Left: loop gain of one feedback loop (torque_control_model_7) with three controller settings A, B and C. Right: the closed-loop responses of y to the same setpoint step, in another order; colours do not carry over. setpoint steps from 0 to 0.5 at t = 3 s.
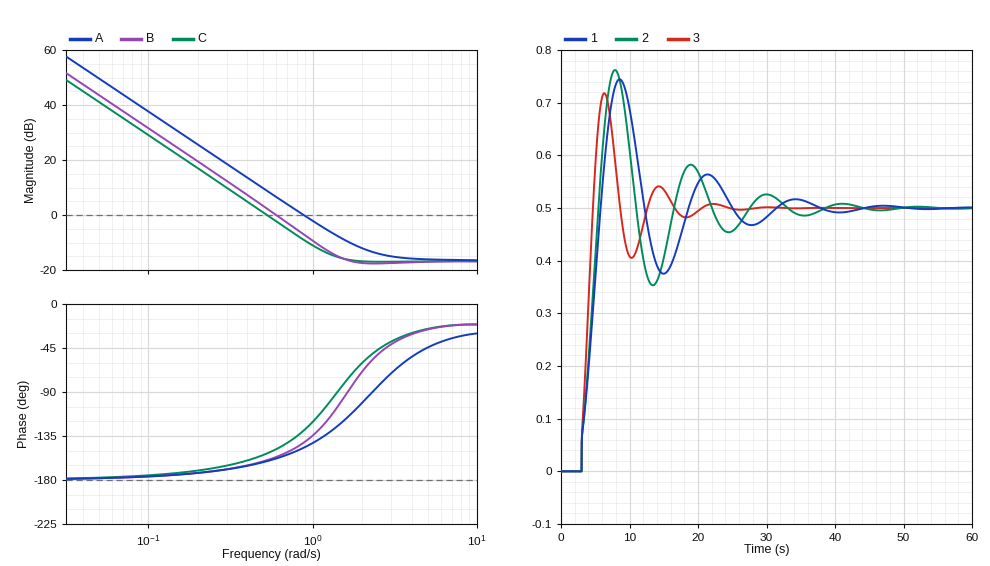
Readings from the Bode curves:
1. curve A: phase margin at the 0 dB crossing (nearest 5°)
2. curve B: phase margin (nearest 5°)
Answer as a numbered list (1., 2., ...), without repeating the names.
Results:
1. 35°
2. 25°
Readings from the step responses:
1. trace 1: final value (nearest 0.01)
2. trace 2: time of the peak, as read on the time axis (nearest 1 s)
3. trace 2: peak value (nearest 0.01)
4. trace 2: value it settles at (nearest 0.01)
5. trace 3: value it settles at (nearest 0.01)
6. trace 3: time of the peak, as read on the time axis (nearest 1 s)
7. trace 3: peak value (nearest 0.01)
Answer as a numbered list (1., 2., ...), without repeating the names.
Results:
1. 0.50
2. 8 s
3. 0.76
4. 0.50
5. 0.50
6. 6 s
7. 0.72
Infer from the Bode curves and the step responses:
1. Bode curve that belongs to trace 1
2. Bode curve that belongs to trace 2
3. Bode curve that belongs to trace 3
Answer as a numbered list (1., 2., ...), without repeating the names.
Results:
1. C
2. B
3. A
